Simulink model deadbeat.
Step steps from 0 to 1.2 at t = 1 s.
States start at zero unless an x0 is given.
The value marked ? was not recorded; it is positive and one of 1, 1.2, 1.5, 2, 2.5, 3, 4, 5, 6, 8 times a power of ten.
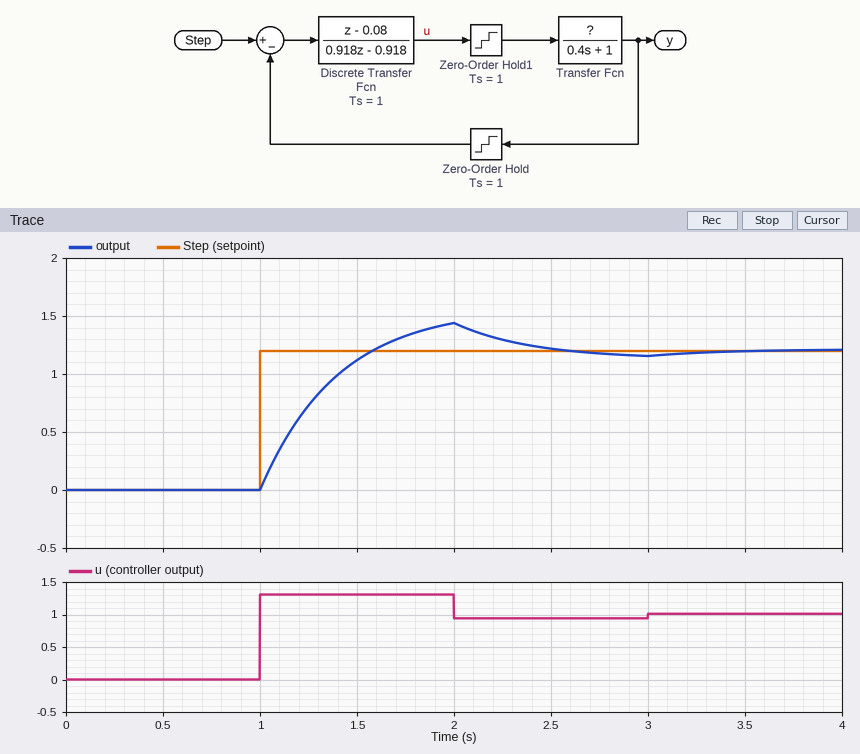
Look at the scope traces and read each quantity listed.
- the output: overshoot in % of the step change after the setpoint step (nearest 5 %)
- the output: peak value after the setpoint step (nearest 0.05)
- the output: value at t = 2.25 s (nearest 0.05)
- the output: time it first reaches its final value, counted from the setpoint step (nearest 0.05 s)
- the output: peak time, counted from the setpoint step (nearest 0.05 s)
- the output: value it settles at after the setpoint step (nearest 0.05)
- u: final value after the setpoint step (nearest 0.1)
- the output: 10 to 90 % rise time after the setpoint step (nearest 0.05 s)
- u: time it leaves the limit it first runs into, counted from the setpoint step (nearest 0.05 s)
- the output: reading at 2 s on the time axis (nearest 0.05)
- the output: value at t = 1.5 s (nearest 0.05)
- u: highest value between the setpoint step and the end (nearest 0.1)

20 %
1.45
1.30
0.60 s
1.00 s
1.20
1.0
0.45 s
1.00 s
1.45
1.10
1.3
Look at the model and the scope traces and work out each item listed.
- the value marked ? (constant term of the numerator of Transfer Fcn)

1.2
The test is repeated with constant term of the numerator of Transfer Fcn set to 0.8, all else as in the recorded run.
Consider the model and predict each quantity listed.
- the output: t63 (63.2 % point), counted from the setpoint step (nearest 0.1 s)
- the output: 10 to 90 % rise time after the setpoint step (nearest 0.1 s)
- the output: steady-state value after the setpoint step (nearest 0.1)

0.5 s
1.3 s
1.2
